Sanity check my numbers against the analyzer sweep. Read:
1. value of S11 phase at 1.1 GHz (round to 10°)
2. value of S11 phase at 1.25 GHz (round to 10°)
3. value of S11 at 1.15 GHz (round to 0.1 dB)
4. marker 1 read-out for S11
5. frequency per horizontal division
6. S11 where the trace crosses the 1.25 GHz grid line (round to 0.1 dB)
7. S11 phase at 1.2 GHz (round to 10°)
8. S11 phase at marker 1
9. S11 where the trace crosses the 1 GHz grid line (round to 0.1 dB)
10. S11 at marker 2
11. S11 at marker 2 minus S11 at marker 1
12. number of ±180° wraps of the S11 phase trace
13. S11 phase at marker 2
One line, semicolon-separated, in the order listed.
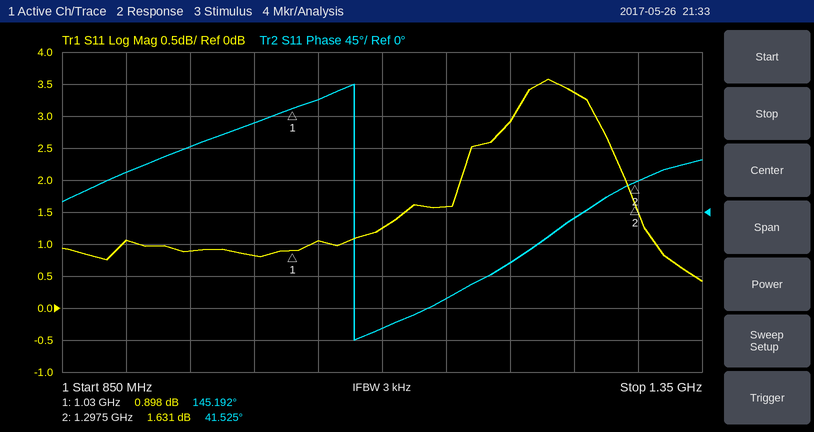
-160°; -10°; 1.6 dB; 0.898 dB; 50 MHz; 3.4 dB; -70°; 145.192°; 0.8 dB; 1.631 dB; 0.733 dB; 1; 41.525°
